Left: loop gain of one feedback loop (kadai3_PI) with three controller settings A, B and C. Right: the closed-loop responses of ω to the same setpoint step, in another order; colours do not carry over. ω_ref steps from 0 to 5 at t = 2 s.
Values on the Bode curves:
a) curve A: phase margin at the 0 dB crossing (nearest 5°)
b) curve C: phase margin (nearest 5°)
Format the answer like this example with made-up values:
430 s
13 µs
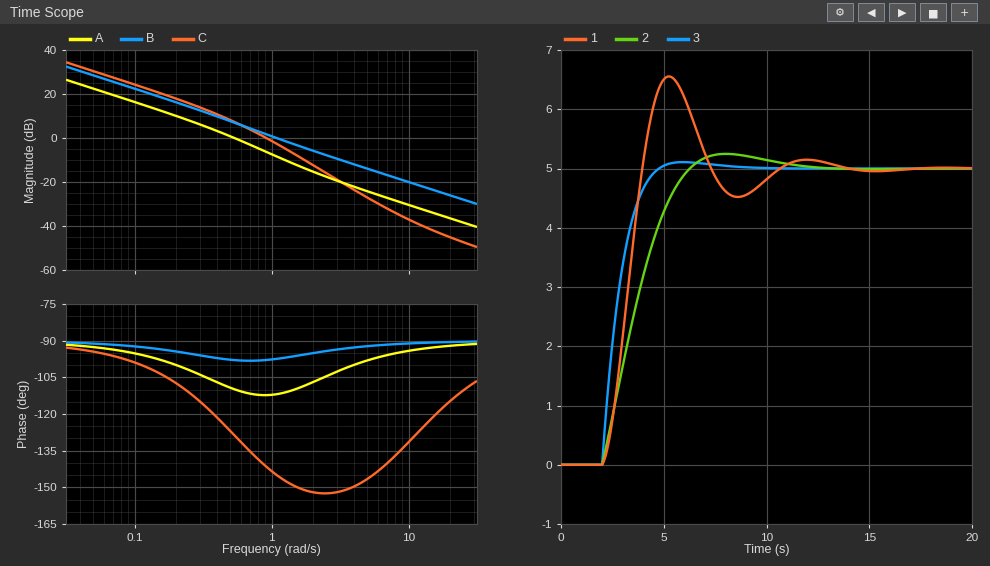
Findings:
70°
40°
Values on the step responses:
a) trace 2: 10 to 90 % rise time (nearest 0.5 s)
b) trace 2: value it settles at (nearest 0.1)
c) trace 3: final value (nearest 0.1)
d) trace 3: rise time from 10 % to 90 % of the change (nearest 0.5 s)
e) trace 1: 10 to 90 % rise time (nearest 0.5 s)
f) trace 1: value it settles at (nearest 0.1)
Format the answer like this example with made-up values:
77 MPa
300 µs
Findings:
3.0 s
5.0
5.0
1.5 s
1.5 s
5.0
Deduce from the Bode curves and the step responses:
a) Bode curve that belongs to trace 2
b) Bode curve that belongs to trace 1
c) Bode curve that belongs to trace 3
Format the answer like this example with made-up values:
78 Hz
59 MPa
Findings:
A
C
B
